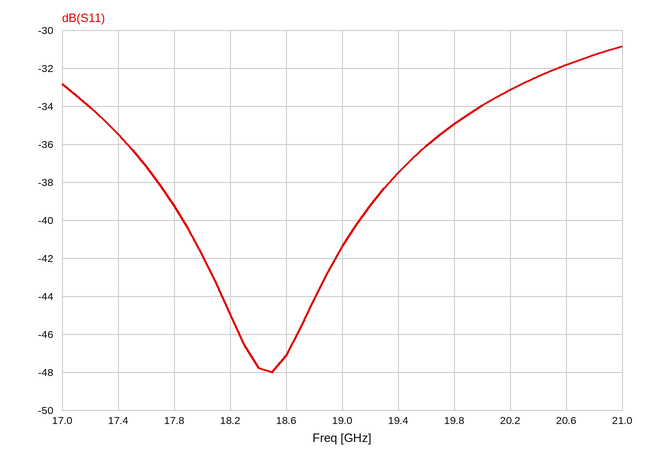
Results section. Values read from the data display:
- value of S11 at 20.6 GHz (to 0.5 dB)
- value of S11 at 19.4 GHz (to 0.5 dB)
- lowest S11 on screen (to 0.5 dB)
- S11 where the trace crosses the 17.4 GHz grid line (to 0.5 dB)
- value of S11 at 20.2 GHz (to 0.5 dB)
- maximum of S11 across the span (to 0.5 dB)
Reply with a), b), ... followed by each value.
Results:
a) -32.0 dB
b) -37.5 dB
c) -48.0 dB
d) -35.5 dB
e) -33.0 dB
f) -31.0 dB
